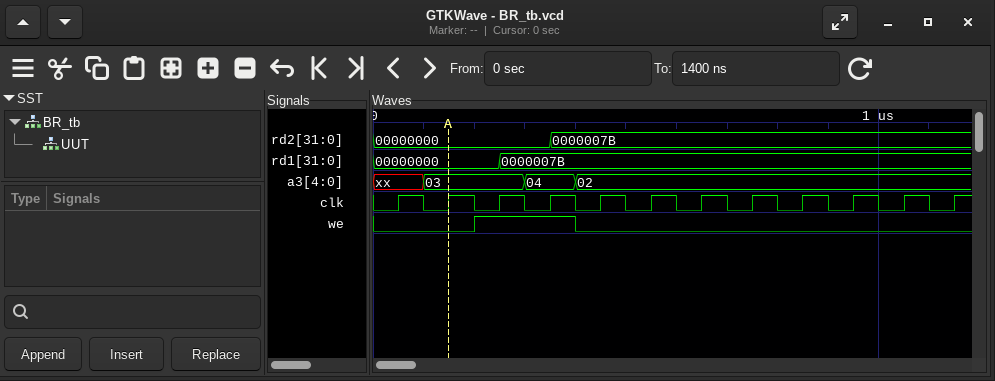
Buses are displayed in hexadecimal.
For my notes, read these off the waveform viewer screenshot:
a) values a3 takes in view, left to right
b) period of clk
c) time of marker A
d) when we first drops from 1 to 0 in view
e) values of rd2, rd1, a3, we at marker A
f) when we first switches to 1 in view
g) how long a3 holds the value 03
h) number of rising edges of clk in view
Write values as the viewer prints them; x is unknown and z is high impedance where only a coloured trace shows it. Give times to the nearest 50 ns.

xx, 03, 04, 02
100 ns
150 ns
400 ns
rd2=00000000, rd1=00000000, a3=03, we=0
200 ns
200 ns
12
